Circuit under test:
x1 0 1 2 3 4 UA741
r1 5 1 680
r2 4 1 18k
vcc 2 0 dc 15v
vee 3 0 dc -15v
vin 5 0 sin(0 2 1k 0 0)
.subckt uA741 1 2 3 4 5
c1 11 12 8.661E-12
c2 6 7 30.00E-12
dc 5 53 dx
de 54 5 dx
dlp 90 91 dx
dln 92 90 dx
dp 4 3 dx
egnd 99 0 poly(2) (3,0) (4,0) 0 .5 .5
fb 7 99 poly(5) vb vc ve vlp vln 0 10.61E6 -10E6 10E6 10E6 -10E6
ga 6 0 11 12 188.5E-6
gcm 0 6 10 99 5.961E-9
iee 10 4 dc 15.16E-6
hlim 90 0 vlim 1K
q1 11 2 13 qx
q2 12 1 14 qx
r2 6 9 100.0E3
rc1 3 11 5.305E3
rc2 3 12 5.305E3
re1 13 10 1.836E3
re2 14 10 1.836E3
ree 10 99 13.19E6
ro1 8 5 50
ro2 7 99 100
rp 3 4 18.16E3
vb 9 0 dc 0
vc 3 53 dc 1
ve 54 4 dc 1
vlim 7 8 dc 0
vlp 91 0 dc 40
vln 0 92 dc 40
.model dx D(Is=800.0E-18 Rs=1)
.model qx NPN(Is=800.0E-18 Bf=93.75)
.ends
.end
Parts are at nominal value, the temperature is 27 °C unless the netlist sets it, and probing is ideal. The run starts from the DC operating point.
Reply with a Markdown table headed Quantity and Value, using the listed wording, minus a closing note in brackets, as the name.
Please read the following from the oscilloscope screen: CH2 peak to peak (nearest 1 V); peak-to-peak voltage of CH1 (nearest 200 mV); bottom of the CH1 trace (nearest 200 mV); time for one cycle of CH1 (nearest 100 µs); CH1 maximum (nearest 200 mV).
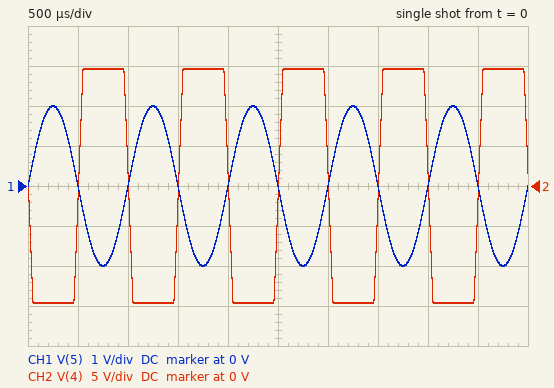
| Quantity | Value |
|---|---|
| CH2 peak to peak | 29 V |
| peak-to-peak voltage of CH1 | 4.0 V |
| bottom of the CH1 trace | -2.0 V |
| time for one cycle of CH1 | 1.0 ms |
| CH1 maximum | 2.0 V |
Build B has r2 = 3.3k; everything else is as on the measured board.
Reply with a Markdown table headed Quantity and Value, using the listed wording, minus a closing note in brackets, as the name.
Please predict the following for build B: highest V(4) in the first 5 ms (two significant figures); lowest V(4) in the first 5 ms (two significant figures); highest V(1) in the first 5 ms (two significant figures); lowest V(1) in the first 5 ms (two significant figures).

| Quantity | Value |
|---|---|
| highest V(4) in the first 5 ms | 9.7 V |
| lowest V(4) in the first 5 ms | -9.7 V |
| highest V(1) in the first 5 ms | 9.9 mV |
| lowest V(1) in the first 5 ms | -9.9 mV |
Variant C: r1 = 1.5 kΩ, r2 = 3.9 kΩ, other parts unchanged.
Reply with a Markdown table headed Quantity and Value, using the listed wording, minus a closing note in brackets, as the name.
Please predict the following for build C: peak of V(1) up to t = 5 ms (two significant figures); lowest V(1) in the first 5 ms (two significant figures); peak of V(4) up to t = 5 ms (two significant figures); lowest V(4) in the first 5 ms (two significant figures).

| Quantity | Value |
|---|---|
| peak of V(1) up to t = 5 ms | 5.3 mV |
| lowest V(1) in the first 5 ms | -5.3 mV |
| peak of V(4) up to t = 5 ms | 5.2 V |
| lowest V(4) in the first 5 ms | -5.2 V |
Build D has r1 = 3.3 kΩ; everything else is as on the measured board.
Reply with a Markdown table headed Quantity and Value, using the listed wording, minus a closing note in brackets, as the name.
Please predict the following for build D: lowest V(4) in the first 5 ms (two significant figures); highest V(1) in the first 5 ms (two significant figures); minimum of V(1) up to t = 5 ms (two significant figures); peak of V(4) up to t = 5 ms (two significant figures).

| Quantity | Value |
|---|---|
| lowest V(4) in the first 5 ms | -11 V |
| highest V(1) in the first 5 ms | 11 mV |
| minimum of V(1) up to t = 5 ms | -11 mV |
| peak of V(4) up to t = 5 ms | 11 V |
